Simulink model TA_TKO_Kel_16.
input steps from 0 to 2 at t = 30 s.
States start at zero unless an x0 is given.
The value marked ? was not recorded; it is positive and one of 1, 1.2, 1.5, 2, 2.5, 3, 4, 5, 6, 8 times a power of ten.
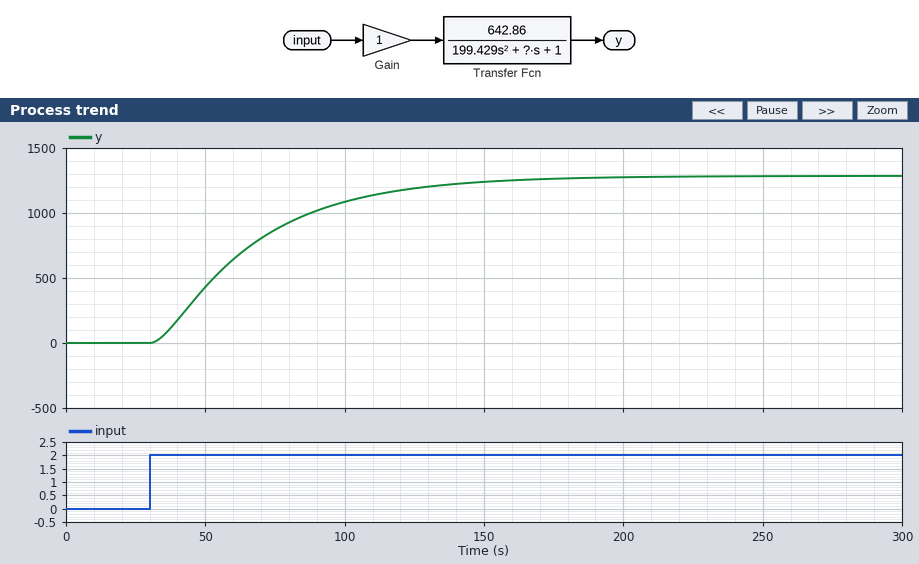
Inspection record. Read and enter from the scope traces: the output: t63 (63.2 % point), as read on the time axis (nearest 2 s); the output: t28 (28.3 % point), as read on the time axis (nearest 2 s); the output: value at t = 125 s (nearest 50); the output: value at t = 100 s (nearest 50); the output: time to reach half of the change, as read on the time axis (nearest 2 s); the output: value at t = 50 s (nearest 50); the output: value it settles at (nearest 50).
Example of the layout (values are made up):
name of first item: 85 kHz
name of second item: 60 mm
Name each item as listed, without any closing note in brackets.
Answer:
the output: t63 (63.2 % point), as read on the time axis: 70 s
the output: t28 (28.3 % point), as read on the time axis: 48 s
the output: value at t = 125 s: 1200
the output: value at t = 100 s: 1100
the output: time to reach half of the change, as read on the time axis: 60 s
the output: value at t = 50 s: 450
the output: value it settles at: 1300
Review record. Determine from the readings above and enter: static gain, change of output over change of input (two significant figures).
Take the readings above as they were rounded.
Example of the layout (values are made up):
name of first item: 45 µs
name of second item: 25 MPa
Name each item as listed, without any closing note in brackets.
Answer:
static gain, change of output over change of input: 650
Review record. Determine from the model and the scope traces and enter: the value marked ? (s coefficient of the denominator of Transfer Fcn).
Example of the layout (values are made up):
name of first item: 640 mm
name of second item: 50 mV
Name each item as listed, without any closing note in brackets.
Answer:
the value marked ?: 40
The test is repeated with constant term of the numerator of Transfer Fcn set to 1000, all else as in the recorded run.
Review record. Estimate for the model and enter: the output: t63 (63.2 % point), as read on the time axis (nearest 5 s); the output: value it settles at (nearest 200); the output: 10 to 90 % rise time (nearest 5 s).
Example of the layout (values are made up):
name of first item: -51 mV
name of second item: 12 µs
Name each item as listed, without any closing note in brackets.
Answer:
the output: t63 (63.2 % point), as read on the time axis: 70 s
the output: value it settles at: 2000
the output: 10 to 90 % rise time: 75 s
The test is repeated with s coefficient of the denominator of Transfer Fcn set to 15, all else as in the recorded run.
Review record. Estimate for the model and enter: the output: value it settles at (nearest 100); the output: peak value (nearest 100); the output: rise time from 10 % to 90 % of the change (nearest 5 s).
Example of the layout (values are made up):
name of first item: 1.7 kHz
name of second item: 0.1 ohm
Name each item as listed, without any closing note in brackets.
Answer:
the output: value it settles at: 1300
the output: peak value: 1500
the output: rise time from 10 % to 90 % of the change: 25 s
